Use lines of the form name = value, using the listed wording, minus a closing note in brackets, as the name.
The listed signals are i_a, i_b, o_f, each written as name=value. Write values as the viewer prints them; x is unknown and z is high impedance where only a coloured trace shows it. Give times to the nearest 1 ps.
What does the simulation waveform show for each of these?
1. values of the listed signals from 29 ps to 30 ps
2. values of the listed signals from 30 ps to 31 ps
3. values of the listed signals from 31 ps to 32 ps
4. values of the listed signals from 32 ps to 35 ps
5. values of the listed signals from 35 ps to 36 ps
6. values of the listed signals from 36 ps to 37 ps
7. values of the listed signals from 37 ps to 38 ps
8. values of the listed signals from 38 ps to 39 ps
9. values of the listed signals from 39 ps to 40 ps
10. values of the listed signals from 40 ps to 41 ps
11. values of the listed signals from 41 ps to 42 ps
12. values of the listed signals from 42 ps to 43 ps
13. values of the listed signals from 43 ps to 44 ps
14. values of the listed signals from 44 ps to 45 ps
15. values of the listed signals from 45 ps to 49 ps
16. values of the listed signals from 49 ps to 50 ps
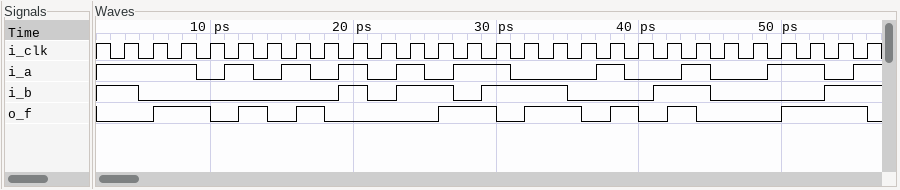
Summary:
values of the listed signals from 29 ps to 30 ps = i_a=1, i_b=1, o_f=1
values of the listed signals from 30 ps to 31 ps = i_a=1, i_b=1, o_f=0
values of the listed signals from 31 ps to 32 ps = i_a=0, i_b=1, o_f=0
values of the listed signals from 32 ps to 35 ps = i_a=0, i_b=1, o_f=1
values of the listed signals from 35 ps to 36 ps = i_a=0, i_b=0, o_f=1
values of the listed signals from 36 ps to 37 ps = i_a=0, i_b=0, o_f=0
values of the listed signals from 37 ps to 38 ps = i_a=1, i_b=0, o_f=0
values of the listed signals from 38 ps to 39 ps = i_a=1, i_b=0, o_f=1
values of the listed signals from 39 ps to 40 ps = i_a=0, i_b=0, o_f=1
values of the listed signals from 40 ps to 41 ps = i_a=0, i_b=0, o_f=0
values of the listed signals from 41 ps to 42 ps = i_a=0, i_b=1, o_f=0
values of the listed signals from 42 ps to 43 ps = i_a=0, i_b=1, o_f=1
values of the listed signals from 43 ps to 44 ps = i_a=1, i_b=1, o_f=1
values of the listed signals from 44 ps to 45 ps = i_a=1, i_b=1, o_f=0
values of the listed signals from 45 ps to 49 ps = i_a=0, i_b=0, o_f=0
values of the listed signals from 49 ps to 50 ps = i_a=1, i_b=0, o_f=0
